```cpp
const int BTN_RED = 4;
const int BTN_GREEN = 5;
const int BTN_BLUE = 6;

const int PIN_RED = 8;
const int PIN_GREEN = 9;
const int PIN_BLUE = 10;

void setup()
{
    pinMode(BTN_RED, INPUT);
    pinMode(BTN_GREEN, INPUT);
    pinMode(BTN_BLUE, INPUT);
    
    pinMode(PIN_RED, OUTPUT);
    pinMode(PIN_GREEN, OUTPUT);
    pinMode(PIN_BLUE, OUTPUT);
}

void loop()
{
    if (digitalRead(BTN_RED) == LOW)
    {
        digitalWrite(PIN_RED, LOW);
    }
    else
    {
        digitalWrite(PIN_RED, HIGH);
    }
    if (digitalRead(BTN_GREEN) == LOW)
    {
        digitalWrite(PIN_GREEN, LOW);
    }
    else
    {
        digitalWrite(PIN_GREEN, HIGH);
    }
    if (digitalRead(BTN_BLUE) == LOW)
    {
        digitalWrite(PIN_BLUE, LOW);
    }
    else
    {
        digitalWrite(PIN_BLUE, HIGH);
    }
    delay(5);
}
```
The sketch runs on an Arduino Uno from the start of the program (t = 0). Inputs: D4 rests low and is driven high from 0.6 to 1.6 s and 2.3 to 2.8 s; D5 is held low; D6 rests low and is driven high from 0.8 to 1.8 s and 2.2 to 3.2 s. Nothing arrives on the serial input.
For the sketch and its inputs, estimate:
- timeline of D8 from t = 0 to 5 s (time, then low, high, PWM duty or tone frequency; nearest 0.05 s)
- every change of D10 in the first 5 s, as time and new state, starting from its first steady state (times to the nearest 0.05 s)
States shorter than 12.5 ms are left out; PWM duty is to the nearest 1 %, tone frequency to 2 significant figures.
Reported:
0 s low; 0.6 s high; 1.6 s low; 2.3 s high; 2.8 s low
0 s low; 0.8 s high; 1.8 s low; 2.2 s high; 3.2 s low
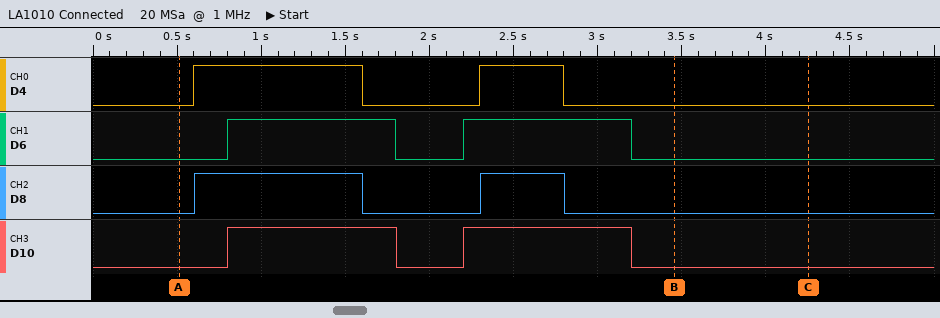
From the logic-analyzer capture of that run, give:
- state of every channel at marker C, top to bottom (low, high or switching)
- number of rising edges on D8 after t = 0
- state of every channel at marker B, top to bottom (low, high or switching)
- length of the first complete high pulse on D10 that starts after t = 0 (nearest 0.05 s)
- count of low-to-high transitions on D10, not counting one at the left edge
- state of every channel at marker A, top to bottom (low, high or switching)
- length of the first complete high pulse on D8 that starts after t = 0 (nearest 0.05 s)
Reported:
D4 low, D6 low, D8 low, D10 low
2
D4 low, D6 low, D8 low, D10 low
1.00 s
2
D4 low, D6 low, D8 low, D10 low
1.00 s
